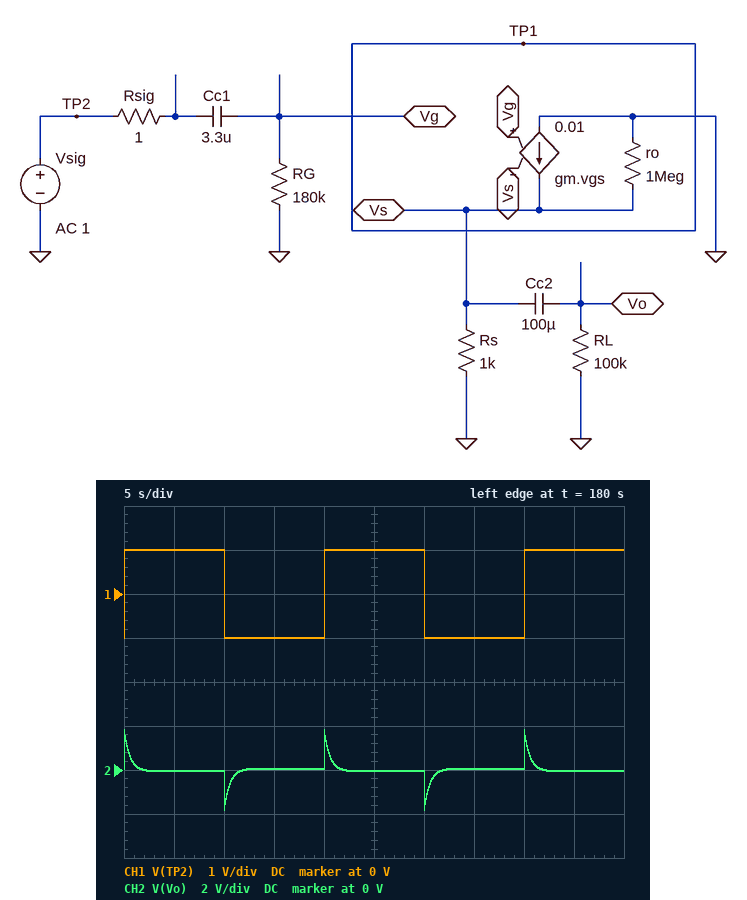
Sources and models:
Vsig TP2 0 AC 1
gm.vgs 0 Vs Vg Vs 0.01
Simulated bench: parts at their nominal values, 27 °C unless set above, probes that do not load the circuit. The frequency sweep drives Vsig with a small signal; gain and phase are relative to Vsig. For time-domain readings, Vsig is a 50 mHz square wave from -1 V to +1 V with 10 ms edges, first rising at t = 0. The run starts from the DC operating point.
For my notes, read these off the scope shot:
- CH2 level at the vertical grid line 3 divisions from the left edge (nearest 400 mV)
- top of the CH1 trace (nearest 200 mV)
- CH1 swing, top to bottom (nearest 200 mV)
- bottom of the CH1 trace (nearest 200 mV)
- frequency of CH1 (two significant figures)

0 V
1.0 V
2.0 V
-1.0 V
50 mHz
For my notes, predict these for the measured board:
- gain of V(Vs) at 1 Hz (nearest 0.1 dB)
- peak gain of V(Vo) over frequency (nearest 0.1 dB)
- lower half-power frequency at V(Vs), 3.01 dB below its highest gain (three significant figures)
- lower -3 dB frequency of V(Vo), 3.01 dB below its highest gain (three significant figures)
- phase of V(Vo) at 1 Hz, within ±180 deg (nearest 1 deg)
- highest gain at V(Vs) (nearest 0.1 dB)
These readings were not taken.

-1.1 dB
-0.8 dB
268 mHz
269 mHz
16 deg
-0.8 dB
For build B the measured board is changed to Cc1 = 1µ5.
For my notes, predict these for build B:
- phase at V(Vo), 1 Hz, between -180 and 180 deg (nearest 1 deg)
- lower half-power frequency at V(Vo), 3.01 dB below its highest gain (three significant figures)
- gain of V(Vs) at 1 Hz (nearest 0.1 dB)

31 deg
590 mHz
-2.1 dB
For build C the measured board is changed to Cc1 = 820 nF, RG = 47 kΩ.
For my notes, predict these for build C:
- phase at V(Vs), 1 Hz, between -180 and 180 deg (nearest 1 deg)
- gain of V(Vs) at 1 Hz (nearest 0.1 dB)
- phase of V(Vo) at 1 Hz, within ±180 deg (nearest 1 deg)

76 deg
-13.4 dB
77 deg
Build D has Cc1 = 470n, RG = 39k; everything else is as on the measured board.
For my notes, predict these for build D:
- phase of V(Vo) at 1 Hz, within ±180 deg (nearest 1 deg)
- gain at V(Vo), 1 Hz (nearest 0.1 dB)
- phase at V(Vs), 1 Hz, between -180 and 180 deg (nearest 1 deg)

84 deg
-19.7 dB
83 deg
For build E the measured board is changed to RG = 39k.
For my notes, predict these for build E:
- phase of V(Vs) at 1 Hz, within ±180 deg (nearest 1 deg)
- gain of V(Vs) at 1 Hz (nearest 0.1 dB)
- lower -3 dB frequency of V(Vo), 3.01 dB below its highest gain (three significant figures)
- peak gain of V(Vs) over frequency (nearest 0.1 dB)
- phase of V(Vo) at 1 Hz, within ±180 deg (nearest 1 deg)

51 deg
-4.9 dB
1.24 Hz
-0.8 dB
52 deg
